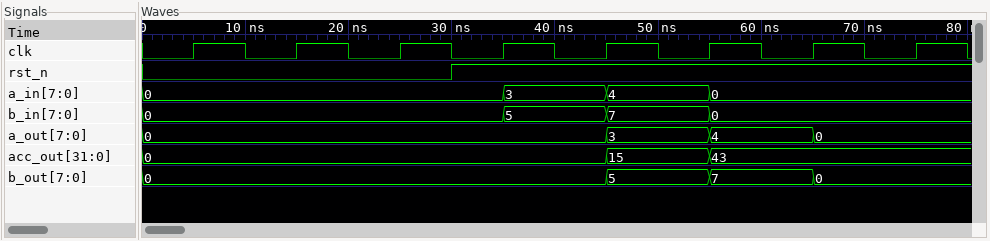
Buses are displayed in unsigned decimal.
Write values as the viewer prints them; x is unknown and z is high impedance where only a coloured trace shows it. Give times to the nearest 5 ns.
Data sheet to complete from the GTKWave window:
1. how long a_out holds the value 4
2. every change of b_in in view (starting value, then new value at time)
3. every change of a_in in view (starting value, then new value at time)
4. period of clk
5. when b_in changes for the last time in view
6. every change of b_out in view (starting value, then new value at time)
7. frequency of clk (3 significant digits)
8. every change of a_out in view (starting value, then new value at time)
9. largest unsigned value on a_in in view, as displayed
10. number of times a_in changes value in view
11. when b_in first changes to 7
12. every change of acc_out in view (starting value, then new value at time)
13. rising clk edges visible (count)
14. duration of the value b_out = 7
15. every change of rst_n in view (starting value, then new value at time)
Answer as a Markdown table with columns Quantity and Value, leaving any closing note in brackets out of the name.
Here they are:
| Quantity | Value |
|---|---|
| how long a_out holds the value 4 | 10 ns |
| every change of b_in in view | 0, 5 at 35 ns, 7 at 45 ns, 0 at 55 ns |
| every change of a_in in view | 0, 3 at 35 ns, 4 at 45 ns, 0 at 55 ns |
| period of clk | 10 ns |
| when b_in changes for the last time in view | 55 ns |
| every change of b_out in view | 0, 5 at 45 ns, 7 at 55 ns, 0 at 65 ns |
| frequency of clk | 100 MHz |
| every change of a_out in view | 0, 3 at 45 ns, 4 at 55 ns, 0 at 65 ns |
| largest unsigned value on a_in in view, as displayed | 4 |
| number of times a_in changes value in view | 3 |
| when b_in first changes to 7 | 45 ns |
| every change of acc_out in view | 0, 15 at 45 ns, 43 at 55 ns |
| rising clk edges visible | 8 |
| duration of the value b_out = 7 | 10 ns |
| every change of rst_n in view | 0, 1 at 30 ns |
